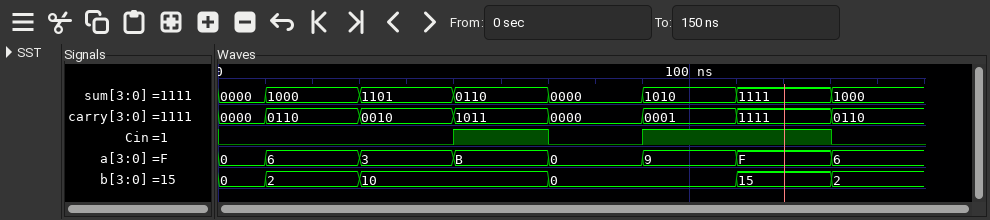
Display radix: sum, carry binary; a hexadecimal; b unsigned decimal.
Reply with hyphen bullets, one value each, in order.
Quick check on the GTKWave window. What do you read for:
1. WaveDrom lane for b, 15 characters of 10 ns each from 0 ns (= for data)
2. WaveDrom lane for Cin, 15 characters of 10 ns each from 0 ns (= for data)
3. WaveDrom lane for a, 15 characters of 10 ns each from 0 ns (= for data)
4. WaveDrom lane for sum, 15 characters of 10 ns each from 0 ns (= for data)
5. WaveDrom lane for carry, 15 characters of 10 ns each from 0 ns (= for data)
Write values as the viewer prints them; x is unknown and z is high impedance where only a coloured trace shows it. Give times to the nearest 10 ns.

- {name: 'b', wave: '==.=...=...=.=.', data: '0 2 10 0 15 2'}
- {name: 'Cin', wave: '0....1.0.1...0.'}
- {name: 'a', wave: '==.=.=.=.=.=.=.', data: '0 6 3 B 0 9 F 6'}
- {name: 'sum', wave: '==.=.=.=.=.=.=.', data: '0000 1000 1101 0110 0000 1010 1111 1000'}
- {name: 'carry', wave: '==.=.=.=.=.=.=.', data: '0000 0110 0010 1011 0000 0001 1111 0110'}
